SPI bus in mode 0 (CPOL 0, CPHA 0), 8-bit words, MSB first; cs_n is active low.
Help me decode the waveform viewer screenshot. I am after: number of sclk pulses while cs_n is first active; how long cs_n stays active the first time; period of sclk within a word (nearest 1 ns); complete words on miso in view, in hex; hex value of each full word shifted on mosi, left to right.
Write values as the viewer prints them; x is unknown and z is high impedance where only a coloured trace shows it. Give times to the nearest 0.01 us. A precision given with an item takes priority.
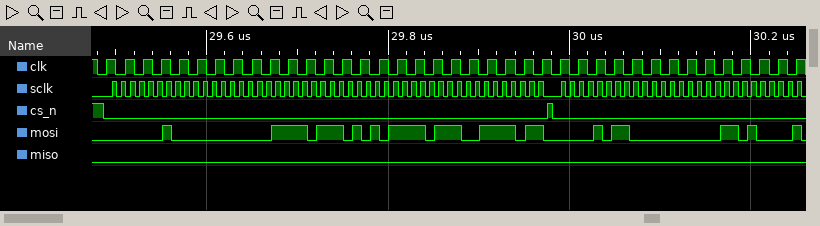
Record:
48
0.49 us
10 ns
00, 00, 00, 00, 00, 00, 00, 00, 00
02, 00, 3D, D5, EE, 7B, 0B, 00, 34
